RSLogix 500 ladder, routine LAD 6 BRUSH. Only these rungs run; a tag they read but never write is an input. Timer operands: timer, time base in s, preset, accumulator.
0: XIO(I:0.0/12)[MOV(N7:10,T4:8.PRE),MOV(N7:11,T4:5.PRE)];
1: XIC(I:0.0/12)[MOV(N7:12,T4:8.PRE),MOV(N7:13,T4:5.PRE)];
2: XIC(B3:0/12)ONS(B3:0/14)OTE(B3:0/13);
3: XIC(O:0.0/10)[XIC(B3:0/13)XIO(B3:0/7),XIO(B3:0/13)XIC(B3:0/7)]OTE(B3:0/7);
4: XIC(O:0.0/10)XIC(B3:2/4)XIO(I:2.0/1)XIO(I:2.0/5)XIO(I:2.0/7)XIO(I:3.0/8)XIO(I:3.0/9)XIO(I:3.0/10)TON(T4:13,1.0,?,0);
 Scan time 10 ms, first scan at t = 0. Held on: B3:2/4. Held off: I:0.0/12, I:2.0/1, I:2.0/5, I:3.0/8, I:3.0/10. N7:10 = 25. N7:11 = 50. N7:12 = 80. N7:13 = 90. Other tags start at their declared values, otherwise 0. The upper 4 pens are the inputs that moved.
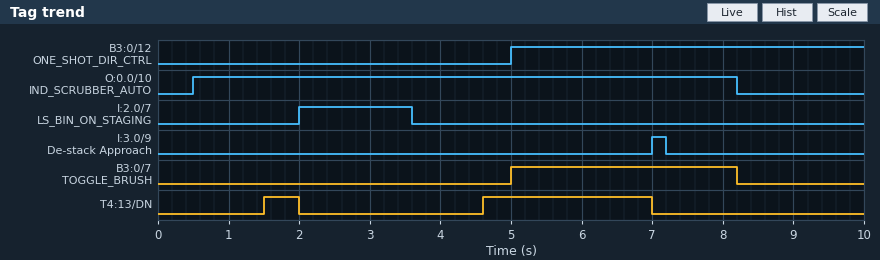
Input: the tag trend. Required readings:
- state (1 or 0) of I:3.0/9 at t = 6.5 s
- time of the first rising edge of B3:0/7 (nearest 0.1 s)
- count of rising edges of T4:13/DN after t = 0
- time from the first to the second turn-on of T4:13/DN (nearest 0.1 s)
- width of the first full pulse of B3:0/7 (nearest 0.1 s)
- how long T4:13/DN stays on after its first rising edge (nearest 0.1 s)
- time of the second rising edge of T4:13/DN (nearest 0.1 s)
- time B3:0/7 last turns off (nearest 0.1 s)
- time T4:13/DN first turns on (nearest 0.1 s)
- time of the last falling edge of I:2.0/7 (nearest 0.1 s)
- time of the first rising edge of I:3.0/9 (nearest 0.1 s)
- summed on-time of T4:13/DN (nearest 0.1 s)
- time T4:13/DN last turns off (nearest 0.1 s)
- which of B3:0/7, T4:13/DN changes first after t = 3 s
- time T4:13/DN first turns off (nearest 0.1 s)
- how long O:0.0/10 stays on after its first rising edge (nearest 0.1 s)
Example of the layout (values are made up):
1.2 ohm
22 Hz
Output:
0
5.0 s
2
3.1 s
3.2 s
0.5 s
4.6 s
8.2 s
1.5 s
3.6 s
7.0 s
2.9 s
7.0 s
T4:13/DN
2.0 s
7.7 s
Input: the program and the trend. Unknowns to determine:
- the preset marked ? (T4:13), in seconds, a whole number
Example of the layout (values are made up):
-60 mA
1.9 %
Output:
1 s
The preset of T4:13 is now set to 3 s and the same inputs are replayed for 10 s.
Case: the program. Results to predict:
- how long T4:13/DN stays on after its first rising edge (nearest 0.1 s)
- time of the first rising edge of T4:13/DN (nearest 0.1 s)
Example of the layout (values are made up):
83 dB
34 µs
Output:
0.4 s
6.6 s
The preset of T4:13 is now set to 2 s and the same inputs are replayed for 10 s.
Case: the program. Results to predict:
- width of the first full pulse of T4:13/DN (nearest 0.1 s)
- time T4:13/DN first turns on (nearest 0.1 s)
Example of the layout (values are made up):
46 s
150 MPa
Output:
1.4 s
5.6 s
